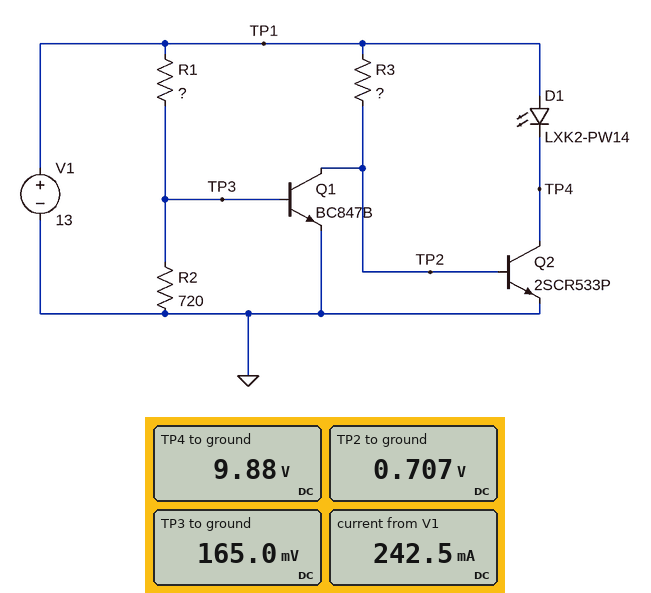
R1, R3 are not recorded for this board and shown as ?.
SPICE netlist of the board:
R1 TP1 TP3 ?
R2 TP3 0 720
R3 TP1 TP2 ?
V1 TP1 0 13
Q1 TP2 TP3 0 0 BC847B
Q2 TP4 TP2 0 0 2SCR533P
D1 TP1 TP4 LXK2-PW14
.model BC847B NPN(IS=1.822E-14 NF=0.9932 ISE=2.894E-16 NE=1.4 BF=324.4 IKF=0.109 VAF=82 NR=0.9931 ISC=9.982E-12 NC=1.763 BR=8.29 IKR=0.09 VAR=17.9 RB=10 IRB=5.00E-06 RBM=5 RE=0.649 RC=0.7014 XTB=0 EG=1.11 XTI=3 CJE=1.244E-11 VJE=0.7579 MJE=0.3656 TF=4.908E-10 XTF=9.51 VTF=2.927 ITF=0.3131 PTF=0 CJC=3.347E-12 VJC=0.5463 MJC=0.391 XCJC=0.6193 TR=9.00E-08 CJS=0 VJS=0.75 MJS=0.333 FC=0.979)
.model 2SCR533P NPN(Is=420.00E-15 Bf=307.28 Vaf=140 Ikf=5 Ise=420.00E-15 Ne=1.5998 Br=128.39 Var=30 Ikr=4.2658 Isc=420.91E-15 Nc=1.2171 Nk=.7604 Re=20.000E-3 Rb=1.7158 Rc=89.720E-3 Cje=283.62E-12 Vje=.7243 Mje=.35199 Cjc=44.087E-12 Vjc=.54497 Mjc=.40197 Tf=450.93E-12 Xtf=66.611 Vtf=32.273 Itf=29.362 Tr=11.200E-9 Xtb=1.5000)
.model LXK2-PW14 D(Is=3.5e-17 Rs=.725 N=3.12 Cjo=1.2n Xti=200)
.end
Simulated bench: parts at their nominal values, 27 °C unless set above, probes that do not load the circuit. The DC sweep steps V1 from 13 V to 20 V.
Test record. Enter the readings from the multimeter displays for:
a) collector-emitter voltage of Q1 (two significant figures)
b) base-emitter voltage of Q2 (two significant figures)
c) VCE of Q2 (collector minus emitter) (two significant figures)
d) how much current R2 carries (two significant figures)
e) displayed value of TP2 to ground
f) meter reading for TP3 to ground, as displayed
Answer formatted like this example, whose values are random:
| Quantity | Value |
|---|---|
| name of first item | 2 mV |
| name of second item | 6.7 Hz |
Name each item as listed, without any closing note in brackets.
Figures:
| Quantity | Value |
|---|---|
| collector-emitter voltage of Q1 | 710 mV |
| base-emitter voltage of Q2 | 710 mV |
| VCE of Q2 (collector minus emitter) | 9.9 V |
| how much current R2 carries | 230 µA |
| displayed value of TP2 to ground | 0.707 V |
| meter reading for TP3 to ground, as displayed | 165.0 mV |
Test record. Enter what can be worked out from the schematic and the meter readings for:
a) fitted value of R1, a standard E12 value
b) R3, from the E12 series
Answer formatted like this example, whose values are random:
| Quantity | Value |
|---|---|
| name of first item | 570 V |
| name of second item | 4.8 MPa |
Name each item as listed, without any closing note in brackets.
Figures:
| Quantity | Value |
|---|---|
| fitted value of R1, a standard E12 value | 56 kΩ |
| R3, from the E12 series | 15 kΩ |
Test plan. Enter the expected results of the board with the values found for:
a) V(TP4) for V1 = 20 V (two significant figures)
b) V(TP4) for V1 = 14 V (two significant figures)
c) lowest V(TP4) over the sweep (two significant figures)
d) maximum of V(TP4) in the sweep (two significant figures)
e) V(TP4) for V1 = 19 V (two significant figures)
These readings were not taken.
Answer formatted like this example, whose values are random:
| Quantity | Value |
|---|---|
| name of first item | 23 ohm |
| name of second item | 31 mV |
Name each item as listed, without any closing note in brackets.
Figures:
| Quantity | Value |
|---|---|
| V(TP4) for V1 = 20 V | 17 V |
| V(TP4) for V1 = 14 V | 11 V |
| lowest V(TP4) over the sweep | 9.9 V |
| maximum of V(TP4) in the sweep | 17 V |
| V(TP4) for V1 = 19 V | 16 V |
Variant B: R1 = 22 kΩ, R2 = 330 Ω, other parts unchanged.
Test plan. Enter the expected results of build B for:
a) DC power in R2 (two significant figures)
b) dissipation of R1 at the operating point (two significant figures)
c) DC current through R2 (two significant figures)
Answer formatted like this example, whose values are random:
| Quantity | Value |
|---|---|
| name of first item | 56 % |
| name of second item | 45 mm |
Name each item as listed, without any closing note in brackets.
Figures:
| Quantity | Value |
|---|---|
| DC power in R2 | 110 µW |
| dissipation of R1 at the operating point | 7.5 mW |
| DC current through R2 | 580 µA |
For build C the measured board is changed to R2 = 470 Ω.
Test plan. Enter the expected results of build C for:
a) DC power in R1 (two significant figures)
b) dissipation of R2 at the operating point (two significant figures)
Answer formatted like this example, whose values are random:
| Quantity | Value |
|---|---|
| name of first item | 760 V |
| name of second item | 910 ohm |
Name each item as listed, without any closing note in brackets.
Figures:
| Quantity | Value |
|---|---|
| DC power in R1 | 3.0 mW |
| dissipation of R2 at the operating point | 25 µW |
